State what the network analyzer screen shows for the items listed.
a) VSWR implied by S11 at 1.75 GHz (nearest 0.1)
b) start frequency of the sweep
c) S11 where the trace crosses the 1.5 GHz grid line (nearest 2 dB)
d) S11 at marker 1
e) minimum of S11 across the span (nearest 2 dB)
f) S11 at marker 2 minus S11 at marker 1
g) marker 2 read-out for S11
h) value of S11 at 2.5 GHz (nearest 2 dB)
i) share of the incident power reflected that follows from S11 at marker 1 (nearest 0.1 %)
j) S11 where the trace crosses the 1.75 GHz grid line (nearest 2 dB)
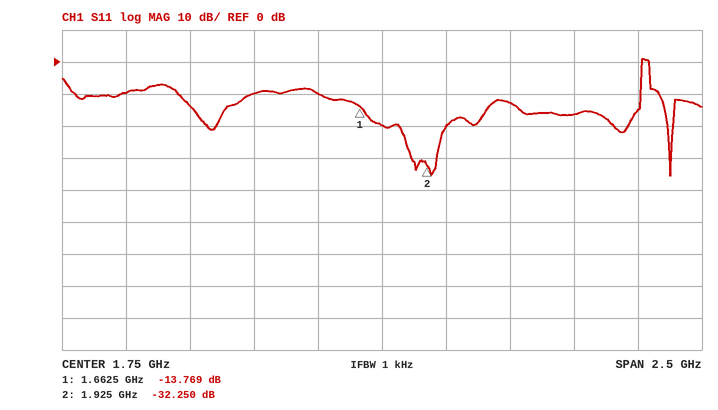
1.2
500 MHz
-10 dB
-13.769 dB
-36 dB
-18.481 dB
-32.250 dB
-16 dB
4.2 %
-20 dB
